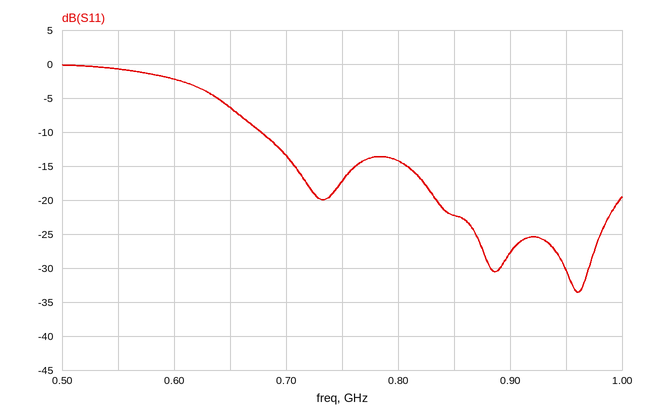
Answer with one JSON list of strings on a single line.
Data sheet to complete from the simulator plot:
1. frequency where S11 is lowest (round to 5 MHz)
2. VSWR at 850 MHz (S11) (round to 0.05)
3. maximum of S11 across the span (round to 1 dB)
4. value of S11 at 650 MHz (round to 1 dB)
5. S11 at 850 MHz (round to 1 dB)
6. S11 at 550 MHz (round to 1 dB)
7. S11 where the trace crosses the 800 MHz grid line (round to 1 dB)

["960 MHz", "1.15", "0 dB", "-6 dB", "-22 dB", "-1 dB", "-14 dB"]
